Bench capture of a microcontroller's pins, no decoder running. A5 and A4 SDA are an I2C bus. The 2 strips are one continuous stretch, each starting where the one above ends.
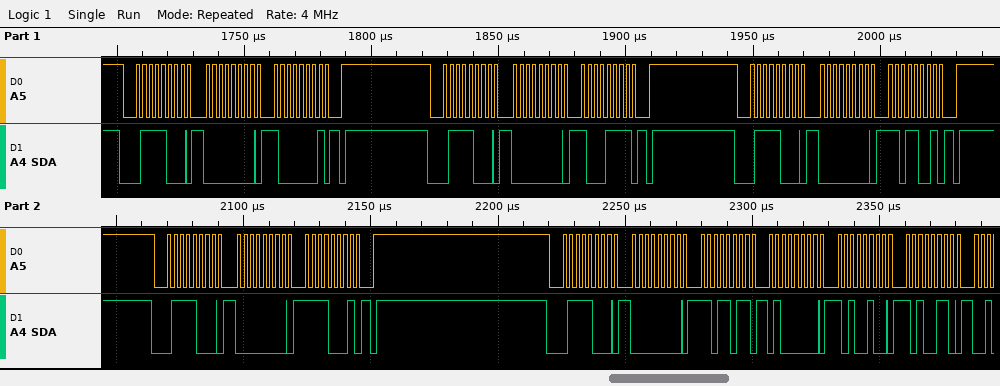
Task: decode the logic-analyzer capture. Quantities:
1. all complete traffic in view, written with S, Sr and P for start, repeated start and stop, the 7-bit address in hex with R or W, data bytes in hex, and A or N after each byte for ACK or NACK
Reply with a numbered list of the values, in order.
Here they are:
1. S 3CW A 00 A 81 A P S 3CW A 00 A 8F A P S 3CW A 00 A D9 A P S 3CW A 00 A F1 A P S 3CW A 00 A DB A 40 A A4 A A6 A
